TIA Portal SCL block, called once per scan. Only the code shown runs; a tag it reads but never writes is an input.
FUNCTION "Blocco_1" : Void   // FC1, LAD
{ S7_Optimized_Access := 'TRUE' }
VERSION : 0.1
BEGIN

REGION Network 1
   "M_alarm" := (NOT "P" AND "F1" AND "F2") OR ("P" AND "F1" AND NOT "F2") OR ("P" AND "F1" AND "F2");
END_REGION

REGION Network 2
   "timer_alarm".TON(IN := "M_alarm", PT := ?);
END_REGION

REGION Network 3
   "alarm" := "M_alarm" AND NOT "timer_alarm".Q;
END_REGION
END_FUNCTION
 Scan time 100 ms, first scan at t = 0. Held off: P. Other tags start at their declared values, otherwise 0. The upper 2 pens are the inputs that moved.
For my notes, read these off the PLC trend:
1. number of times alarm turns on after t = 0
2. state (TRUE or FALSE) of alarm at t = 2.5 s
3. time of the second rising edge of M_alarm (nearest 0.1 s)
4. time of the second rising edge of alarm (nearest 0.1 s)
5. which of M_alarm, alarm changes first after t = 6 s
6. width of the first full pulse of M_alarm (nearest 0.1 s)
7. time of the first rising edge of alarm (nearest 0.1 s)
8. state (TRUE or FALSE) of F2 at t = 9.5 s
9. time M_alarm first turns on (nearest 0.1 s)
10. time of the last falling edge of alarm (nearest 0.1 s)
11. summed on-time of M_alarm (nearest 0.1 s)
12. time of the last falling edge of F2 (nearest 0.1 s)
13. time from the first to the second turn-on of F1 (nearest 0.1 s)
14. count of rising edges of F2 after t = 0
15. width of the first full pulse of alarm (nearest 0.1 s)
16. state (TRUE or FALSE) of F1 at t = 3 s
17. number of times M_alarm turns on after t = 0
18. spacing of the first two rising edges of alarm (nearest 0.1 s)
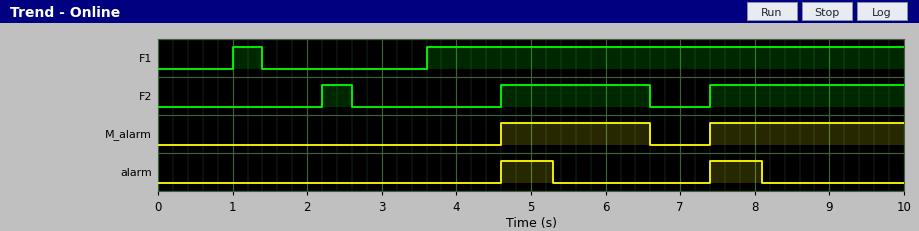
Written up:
2
FALSE
7.4 s
7.4 s
M_alarm
2.0 s
4.6 s
TRUE
4.6 s
8.1 s
4.6 s
6.6 s
2.6 s
3
0.7 s
FALSE
2
2.8 s
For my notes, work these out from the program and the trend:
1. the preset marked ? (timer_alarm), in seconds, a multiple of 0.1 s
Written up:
0.7 s
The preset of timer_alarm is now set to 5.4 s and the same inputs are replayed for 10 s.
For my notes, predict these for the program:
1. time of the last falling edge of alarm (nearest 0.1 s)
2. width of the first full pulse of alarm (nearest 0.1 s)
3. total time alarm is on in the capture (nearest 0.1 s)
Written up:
6.6 s
2.0 s
4.6 s
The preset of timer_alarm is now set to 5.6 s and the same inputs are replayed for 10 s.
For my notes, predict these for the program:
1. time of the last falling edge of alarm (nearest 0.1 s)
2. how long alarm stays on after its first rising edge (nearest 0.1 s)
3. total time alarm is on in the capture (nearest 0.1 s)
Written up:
6.6 s
2.0 s
4.6 s
